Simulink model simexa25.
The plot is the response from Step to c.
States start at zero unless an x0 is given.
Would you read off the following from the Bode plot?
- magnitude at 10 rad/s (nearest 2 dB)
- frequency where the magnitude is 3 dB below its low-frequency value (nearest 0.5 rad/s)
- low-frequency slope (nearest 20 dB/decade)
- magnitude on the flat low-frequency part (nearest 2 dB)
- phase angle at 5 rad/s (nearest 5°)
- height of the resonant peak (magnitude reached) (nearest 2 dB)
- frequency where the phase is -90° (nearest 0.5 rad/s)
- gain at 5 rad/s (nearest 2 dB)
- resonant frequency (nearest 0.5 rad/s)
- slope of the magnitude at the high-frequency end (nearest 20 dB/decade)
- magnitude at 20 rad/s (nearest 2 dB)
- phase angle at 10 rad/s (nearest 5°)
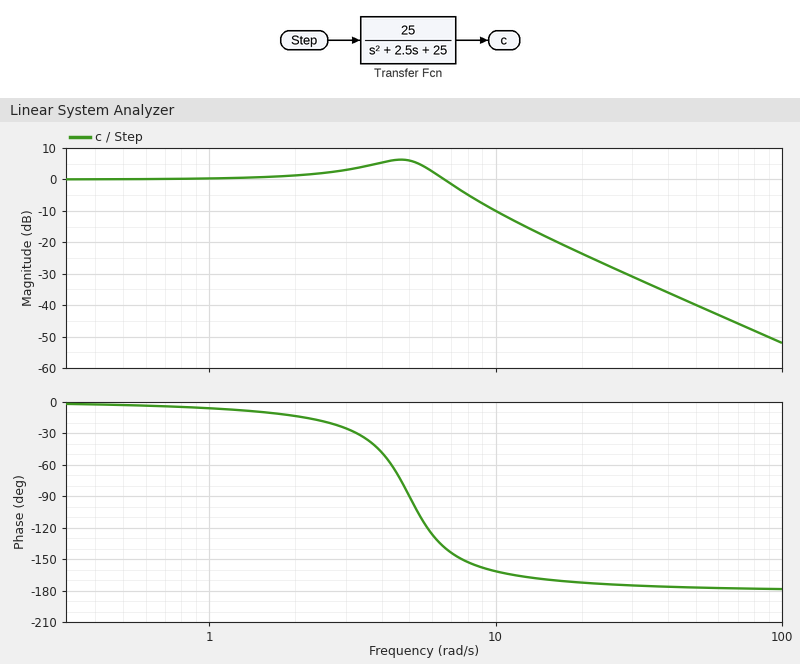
-10 dB
7.5 rad/s
0 dB/decade
0 dB
-90°
6 dB
5.0 rad/s
6 dB
4.5 rad/s
-40 dB/decade
-24 dB
-160°
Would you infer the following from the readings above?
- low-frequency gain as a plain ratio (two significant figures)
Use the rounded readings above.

1.0
